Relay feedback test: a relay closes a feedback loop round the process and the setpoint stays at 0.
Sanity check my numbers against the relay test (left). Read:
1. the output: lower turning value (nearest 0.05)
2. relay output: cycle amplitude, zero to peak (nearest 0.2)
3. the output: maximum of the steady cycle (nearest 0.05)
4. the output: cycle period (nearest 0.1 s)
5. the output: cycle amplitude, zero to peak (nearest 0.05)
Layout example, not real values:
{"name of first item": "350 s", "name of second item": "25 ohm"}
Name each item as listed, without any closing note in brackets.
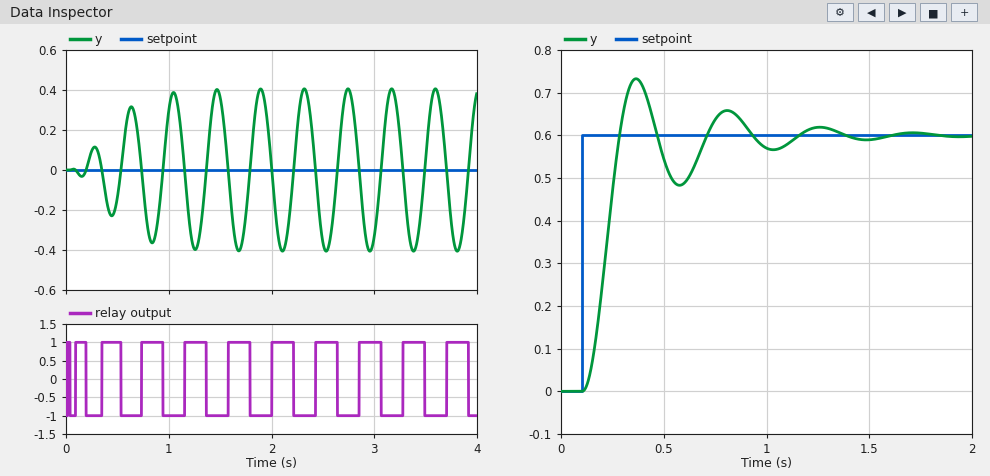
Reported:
{"the output: lower turning value": "-0.40", "relay output: cycle amplitude, zero to peak": "1.0", "the output: maximum of the steady cycle": "0.40", "the output: cycle period": "0.4 s", "the output: cycle amplitude, zero to peak": "0.40"}
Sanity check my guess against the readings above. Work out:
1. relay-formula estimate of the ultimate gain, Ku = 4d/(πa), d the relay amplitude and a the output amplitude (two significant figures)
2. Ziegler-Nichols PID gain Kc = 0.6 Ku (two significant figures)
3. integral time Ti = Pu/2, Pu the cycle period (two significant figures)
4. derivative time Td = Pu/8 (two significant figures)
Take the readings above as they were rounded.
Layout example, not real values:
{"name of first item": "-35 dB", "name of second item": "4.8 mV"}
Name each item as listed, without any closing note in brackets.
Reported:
{"relay-formula estimate of the ultimate gain, Ku = 4d/(πa), d the relay amplitude and a the output amplitude": "3.2", "Ziegler-Nichols PID gain Kc = 0.6 Ku": "1.9", "integral time Ti = Pu/2, Pu the cycle period": "0.20 s", "derivative time Td = Pu/8": "0.050 s"}
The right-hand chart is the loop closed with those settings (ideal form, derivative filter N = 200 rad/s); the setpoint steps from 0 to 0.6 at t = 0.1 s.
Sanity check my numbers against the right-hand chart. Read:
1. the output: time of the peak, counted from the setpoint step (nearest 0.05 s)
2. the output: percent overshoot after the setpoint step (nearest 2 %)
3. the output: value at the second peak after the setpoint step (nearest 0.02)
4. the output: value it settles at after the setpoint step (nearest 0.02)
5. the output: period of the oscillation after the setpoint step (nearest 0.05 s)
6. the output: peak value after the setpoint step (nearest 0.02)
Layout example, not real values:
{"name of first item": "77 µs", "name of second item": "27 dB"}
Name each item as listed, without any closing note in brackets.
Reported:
{"the output: time of the peak, counted from the setpoint step": "0.25 s", "the output: percent overshoot after the setpoint step": "22 %", "the output: value at the second peak after the setpoint step": "0.66", "the output: value it settles at after the setpoint step": "0.60", "the output: period of the oscillation after the setpoint step": "0.45 s", "the output: peak value after the setpoint step": "0.74"}
